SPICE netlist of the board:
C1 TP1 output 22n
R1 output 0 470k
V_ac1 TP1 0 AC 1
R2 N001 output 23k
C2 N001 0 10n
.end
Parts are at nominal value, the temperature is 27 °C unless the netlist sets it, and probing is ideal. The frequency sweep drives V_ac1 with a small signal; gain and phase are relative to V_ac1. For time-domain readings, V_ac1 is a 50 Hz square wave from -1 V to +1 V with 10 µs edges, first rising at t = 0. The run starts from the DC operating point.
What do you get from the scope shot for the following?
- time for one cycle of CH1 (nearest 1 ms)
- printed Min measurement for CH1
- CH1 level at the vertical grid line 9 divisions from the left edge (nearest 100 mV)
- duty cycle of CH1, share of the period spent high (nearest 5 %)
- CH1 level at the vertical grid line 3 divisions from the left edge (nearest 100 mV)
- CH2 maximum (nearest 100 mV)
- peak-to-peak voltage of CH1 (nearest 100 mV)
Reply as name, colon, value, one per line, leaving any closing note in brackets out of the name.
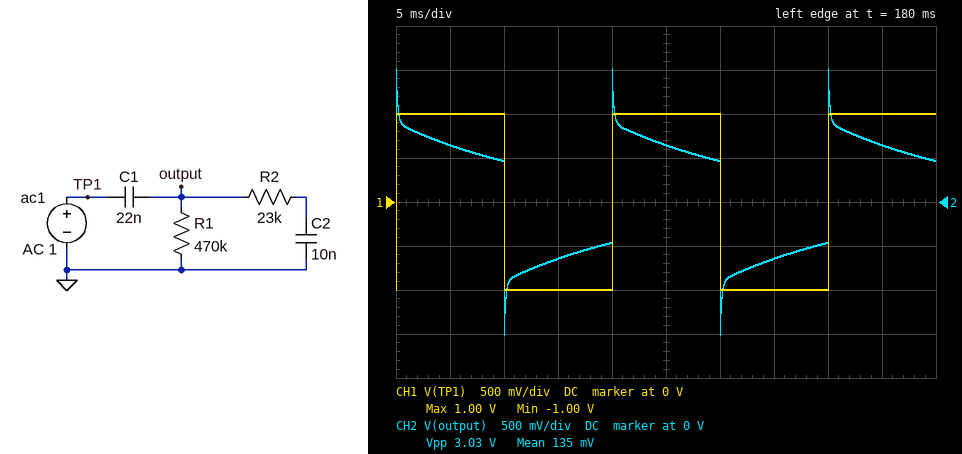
time for one cycle of CH1: 20 ms
printed Min measurement for CH1: -1.00 V
CH1 level at the vertical grid line 9 divisions from the left edge: 1.0 V
duty cycle of CH1, share of the period spent high: 50 %
CH1 level at the vertical grid line 3 divisions from the left edge: -1.0 V
CH2 maximum: 1.5 V
peak-to-peak voltage of CH1: 2.0 V
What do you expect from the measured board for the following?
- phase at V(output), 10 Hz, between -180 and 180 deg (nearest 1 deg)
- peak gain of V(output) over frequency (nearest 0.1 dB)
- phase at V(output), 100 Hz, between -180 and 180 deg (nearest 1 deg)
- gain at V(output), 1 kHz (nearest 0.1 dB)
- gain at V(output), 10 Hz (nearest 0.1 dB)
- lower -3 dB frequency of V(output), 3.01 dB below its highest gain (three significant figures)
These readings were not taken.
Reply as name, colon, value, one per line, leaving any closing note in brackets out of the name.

phase at V(output), 10 Hz, between -180 and 180 deg: 47 deg
peak gain of V(output) over frequency: 0 dB
phase at V(output), 100 Hz, between -180 and 180 deg: 9 deg
gain at V(output), 1 kHz: -1.4 dB
gain at V(output), 10 Hz: -6.5 dB
lower -3 dB frequency of V(output), 3.01 dB below its highest gain: 259 Hz
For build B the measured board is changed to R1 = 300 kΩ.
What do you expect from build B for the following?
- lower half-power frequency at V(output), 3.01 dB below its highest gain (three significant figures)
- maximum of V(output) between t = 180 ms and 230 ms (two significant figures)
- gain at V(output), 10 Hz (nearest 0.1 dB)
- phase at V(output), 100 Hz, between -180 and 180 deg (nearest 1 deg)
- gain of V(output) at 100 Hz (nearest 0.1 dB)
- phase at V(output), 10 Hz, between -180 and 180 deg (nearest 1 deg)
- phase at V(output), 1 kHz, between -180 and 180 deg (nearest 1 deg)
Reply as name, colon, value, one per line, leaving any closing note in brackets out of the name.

lower half-power frequency at V(output), 3.01 dB below its highest gain: 274 Hz
maximum of V(output) between t = 180 ms and 230 ms: 1.6 V
gain at V(output), 10 Hz: -9.0 dB
phase at V(output), 100 Hz, between -180 and 180 deg: 12 deg
gain of V(output) at 100 Hz: -3.4 dB
phase at V(output), 10 Hz, between -180 and 180 deg: 59 deg
phase at V(output), 1 kHz, between -180 and 180 deg: 12 deg
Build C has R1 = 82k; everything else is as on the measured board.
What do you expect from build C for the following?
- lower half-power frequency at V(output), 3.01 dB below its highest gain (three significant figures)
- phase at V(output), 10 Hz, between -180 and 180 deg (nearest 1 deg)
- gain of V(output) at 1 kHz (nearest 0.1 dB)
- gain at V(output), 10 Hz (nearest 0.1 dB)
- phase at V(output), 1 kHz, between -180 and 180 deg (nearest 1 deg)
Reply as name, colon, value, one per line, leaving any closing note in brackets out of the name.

lower half-power frequency at V(output), 3.01 dB below its highest gain: 380 Hz
phase at V(output), 10 Hz, between -180 and 180 deg: 81 deg
gain of V(output) at 1 kHz: -1.5 dB
gain at V(output), 10 Hz: -19.0 dB
phase at V(output), 1 kHz, between -180 and 180 deg: 15 deg
